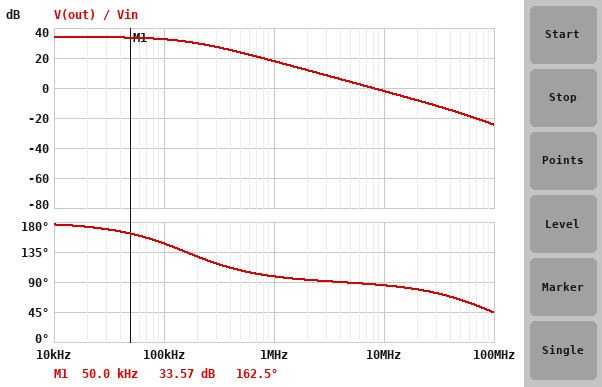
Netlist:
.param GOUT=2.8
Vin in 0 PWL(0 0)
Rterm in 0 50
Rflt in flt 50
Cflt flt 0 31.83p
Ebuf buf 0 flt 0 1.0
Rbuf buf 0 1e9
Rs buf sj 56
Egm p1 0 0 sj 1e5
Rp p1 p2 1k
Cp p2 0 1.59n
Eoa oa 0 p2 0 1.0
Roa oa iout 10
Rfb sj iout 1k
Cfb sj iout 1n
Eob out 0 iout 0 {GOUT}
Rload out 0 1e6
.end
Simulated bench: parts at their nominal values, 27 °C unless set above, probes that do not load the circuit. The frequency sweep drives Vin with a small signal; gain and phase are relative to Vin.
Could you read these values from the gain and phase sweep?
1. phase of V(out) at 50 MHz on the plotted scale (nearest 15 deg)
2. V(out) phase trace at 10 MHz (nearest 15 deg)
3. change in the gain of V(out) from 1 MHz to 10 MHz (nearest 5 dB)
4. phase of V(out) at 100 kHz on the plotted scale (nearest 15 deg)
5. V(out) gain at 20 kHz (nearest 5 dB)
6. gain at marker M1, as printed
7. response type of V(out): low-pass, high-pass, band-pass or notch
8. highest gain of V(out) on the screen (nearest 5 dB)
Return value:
60 deg
90 deg
-20 dB
150 deg
35 dB
33.57 dB
low-pass
35 dB
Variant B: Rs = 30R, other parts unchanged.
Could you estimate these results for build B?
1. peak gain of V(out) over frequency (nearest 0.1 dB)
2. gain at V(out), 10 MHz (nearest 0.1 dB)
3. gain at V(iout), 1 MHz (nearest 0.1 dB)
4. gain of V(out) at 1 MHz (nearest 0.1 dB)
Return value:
39.4 dB
3.4 dB
14.4 dB
23.3 dB
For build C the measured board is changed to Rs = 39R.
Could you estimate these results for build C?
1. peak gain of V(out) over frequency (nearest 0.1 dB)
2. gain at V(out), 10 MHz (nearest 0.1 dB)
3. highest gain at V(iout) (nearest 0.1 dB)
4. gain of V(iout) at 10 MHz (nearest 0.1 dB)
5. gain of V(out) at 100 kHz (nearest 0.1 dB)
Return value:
37.1 dB
1.1 dB
28.2 dB
-7.8 dB
35.7 dB
